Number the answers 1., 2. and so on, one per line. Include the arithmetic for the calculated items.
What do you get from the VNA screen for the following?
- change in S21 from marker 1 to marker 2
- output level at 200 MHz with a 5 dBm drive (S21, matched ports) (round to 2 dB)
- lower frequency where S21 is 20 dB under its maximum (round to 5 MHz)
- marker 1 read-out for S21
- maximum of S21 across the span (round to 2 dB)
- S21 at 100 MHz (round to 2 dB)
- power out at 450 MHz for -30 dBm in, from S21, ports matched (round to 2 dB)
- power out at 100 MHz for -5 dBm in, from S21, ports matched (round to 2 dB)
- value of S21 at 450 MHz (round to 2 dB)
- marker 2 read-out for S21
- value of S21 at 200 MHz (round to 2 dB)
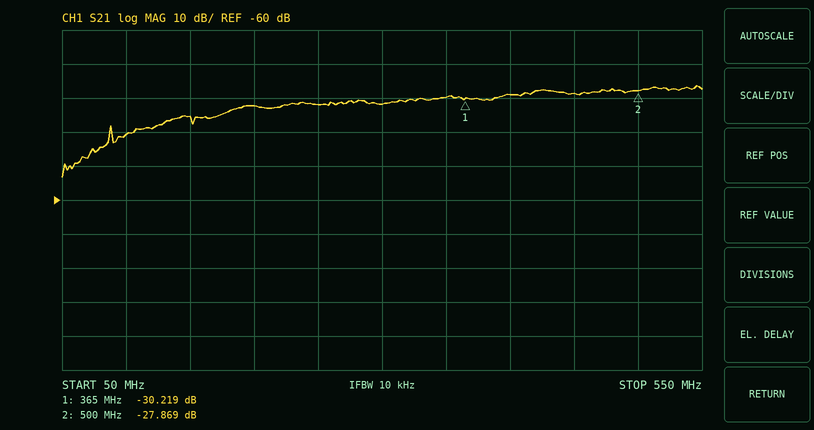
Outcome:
1. -27.869 − (-30.219) = 2.350 dB
2. 5 dBm + (-32 dB) = -28 dBm
3. 70 MHz
4. -30.219 dB
5. -26 dB
6. -40 dB
7. -30 dBm + (-28 dB) = -58 dBm
8. -5 dBm + (-40 dB) = -46 dBm
9. -28 dB
10. -27.869 dB
11. -32 dB
